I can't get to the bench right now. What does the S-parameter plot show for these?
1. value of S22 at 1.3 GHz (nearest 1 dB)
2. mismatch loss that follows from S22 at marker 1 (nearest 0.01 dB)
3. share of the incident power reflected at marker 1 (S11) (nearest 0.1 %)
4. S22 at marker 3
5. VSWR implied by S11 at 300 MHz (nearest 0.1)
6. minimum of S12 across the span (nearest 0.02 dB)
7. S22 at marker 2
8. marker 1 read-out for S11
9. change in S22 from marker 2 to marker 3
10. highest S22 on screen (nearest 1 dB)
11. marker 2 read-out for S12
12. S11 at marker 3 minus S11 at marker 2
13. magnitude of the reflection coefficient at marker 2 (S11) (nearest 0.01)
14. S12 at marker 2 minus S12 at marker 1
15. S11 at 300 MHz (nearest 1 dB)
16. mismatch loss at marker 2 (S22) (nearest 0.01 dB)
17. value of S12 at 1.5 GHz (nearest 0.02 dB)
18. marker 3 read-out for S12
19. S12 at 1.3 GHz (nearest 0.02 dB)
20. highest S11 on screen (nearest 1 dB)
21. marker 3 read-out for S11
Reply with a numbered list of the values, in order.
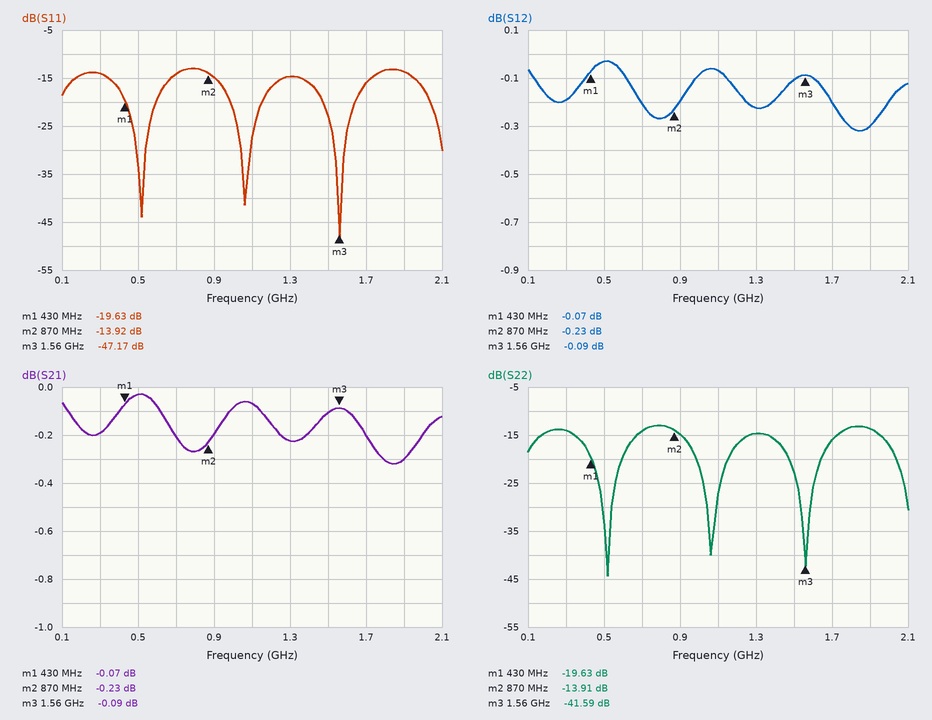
1. -15 dB
2. 0.05 dB
3. 1.1 %
4. -41.59 dB
5. 1.5
6. -0.32 dB
7. -13.91 dB
8. -19.63 dB
9. -27.68 dB
10. -13 dB
11. -0.23 dB
12. -33.25 dB
13. 0.20
14. -0.16 dB
15. -14 dB
16. 0.18 dB
17. -0.10 dB
18. -0.09 dB
19. -0.22 dB
20. -13 dB
21. -47.17 dB
